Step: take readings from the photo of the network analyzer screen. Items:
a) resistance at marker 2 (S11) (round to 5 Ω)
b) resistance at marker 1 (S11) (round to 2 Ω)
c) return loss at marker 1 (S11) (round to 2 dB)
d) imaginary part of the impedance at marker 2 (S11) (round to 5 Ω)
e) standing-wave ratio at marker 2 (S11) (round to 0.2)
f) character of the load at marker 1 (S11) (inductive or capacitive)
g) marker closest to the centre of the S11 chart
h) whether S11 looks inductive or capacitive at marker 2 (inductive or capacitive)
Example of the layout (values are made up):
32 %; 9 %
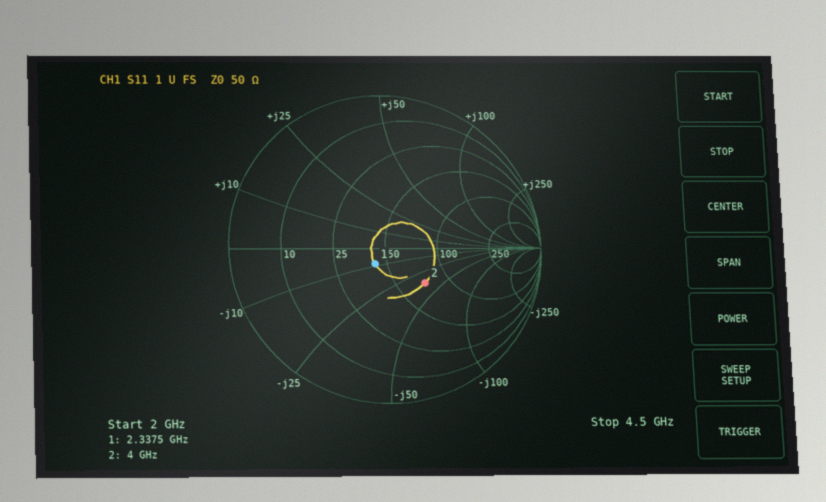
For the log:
70 Ω; 42 Ω; 18 dB; -35 Ω; 2.0; capacitive; marker 1; capacitive
